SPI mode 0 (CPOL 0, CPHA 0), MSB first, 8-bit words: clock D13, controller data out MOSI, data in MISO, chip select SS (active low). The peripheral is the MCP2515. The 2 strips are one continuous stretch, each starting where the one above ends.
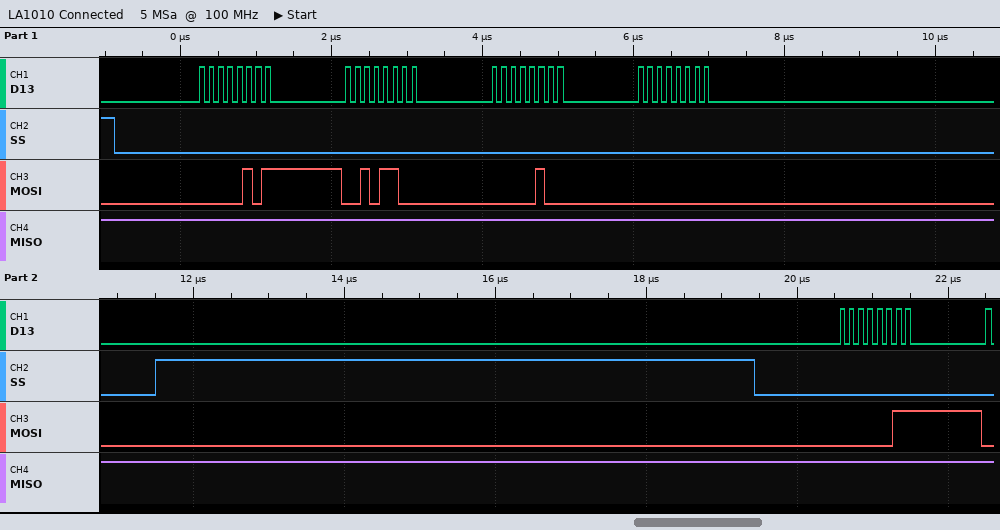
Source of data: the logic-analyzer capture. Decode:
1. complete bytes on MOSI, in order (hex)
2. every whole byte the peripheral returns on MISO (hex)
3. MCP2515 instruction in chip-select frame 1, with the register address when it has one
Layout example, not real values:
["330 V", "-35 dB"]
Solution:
["05 2C 04 00 03", "FF FF FF FF FF", "BIT MODIFY 0x2C"]
